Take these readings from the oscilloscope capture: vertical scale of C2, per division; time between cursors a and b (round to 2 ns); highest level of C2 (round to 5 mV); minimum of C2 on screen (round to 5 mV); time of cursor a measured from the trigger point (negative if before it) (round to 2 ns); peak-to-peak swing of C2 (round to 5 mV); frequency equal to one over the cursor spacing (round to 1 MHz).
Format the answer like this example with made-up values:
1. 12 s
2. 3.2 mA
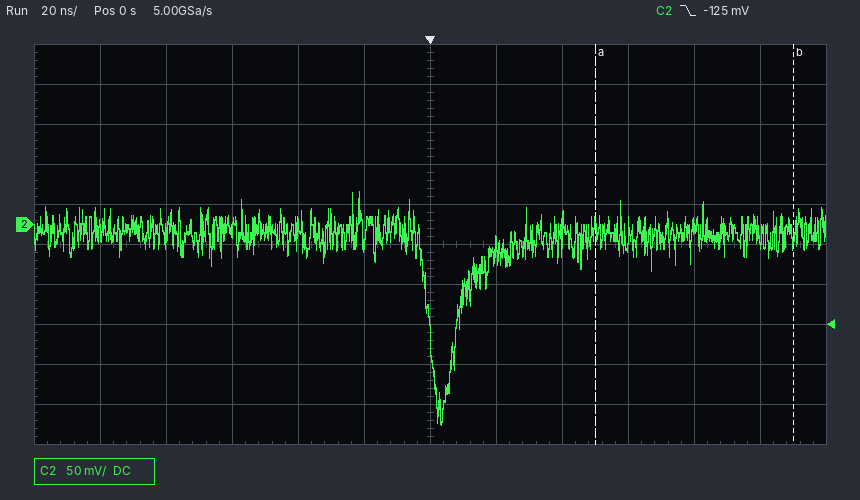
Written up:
1. 50 mV
2. 60 ns
3. 40 mV
4. -250 mV
5. +50 ns
6. 290 mV
7. 17 MHz
